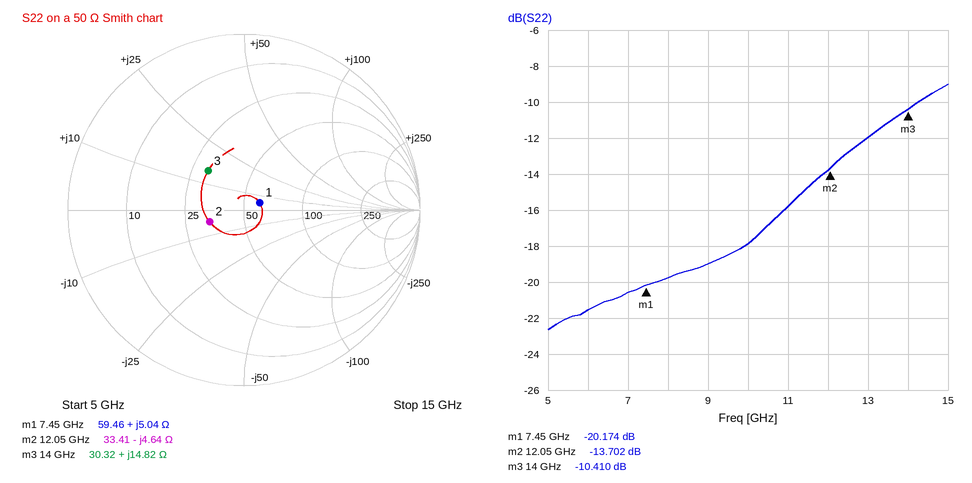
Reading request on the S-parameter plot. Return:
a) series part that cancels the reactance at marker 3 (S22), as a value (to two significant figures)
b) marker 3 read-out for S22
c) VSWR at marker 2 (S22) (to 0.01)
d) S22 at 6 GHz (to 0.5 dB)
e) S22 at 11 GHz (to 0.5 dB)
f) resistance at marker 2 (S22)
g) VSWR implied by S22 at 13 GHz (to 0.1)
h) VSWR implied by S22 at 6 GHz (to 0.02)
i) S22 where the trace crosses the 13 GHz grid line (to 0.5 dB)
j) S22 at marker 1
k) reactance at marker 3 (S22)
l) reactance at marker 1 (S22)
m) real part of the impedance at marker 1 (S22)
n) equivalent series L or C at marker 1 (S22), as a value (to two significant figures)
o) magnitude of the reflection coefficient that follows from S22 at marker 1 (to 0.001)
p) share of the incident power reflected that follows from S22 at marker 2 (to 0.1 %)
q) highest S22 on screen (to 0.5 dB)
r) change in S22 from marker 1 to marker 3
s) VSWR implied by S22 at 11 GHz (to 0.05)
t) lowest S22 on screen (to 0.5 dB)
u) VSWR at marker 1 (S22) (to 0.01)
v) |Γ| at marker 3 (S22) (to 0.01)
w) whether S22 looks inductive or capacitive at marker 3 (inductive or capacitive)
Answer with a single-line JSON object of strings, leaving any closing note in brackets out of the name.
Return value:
{"series part that cancels the reactance at marker 3 (S22), as a value": "770 fF", "marker 3 read-out for S22": "-10.410 dB", "VSWR at marker 2 (S22)": "1.52", "S22 at 6 GHz": "-21.5 dB", "S22 at 11 GHz": "-16.0 dB", "resistance at marker 2": "33.41 Ω", "VSWR implied by S22 at 13 GHz": "1.7", "VSWR implied by S22 at 6 GHz": "1.18", "S22 where the trace crosses the 13 GHz grid line": "-12.0 dB", "S22 at marker 1": "-20.174 dB", "reactance at marker 3": "+14.82 Ω", "reactance at marker 1": "+5.04 Ω", "real part of the impedance at marker 1": "59.46 Ω", "equivalent series L or C at marker 1 (S22), as a value": "110 pH", "magnitude of the reflection coefficient that follows from S22 at marker 1": "0.098", "share of the incident power reflected that follows from S22 at marker 2": "4.3 %", "highest S22 on screen": "-9.0 dB", "change in S22 from marker 1 to marker 3": "9.764 dB", "VSWR implied by S22 at 11 GHz": "1.40", "lowest S22 on screen": "-22.5 dB", "VSWR at marker 1 (S22)": "1.22", "|Γ| at marker 3 (S22)": "0.30", "whether S22 looks inductive or capacitive at marker 3": "inductive"}
